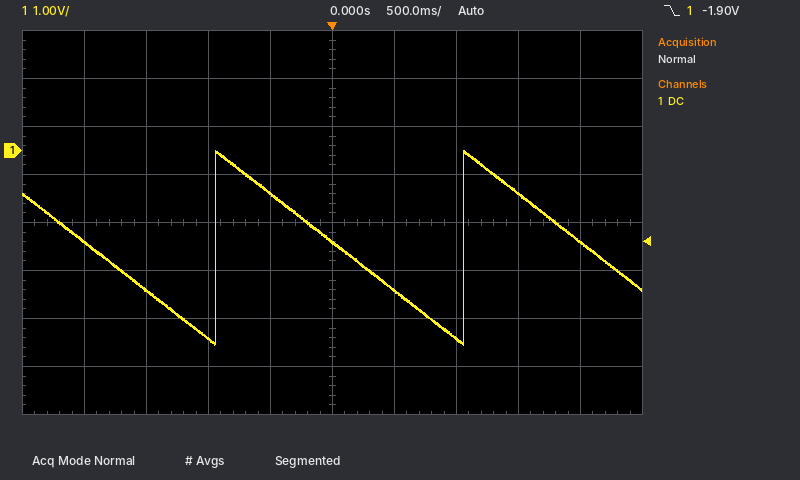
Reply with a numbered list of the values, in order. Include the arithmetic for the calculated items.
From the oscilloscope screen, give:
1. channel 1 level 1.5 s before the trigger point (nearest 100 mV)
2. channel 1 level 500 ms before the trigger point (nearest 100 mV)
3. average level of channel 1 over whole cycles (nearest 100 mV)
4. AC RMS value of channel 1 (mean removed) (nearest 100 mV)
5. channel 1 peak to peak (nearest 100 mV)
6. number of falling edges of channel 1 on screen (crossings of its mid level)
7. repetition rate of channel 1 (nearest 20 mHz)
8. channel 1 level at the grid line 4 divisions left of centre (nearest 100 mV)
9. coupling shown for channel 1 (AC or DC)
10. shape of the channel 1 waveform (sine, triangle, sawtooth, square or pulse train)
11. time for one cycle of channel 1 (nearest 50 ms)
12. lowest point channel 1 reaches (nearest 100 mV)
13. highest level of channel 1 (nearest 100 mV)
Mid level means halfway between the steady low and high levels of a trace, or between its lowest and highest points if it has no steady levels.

1. -2.9 V
2. -900 mV
3. (0.0 V + (-4.1 V)) / 2 ≈ -2.0 V
4. 4.1 V / (2√3) ≈ 1.2 V
5. 0.0 V − (-4.1 V) = 4.1 V
6. 3
7. 1 / 2.00 s ≈ 500 mHz
8. -1.9 V
9. DC
10. sawtooth
11. 2.00 s
12. -4.1 V
13. 0.0 V
